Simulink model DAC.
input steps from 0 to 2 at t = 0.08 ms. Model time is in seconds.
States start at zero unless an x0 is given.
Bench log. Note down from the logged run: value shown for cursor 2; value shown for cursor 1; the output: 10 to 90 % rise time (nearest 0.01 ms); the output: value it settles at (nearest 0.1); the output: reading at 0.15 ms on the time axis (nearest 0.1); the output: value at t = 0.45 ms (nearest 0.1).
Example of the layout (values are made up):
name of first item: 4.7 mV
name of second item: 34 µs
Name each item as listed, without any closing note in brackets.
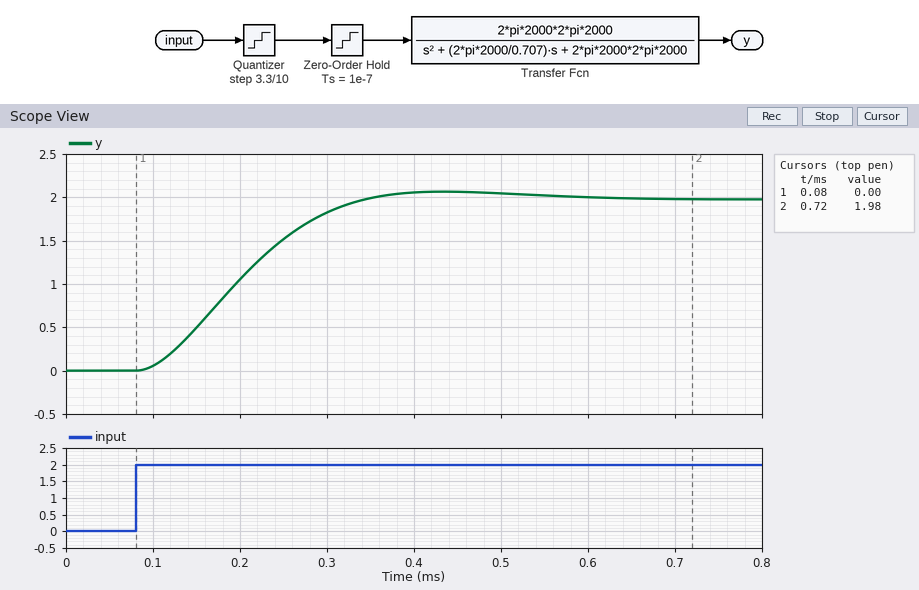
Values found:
value shown for cursor 2: 1.98
value shown for cursor 1: 0.00
the output: 10 to 90 % rise time: 0.17 ms
the output: value it settles at: 2.0
the output: reading at 0.15 ms on the time axis: 0.5
the output: value at t = 0.45 ms: 2.1
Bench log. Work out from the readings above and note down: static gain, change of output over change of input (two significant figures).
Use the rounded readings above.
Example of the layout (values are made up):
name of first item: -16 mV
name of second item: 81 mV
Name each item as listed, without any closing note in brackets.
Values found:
static gain, change of output over change of input: 1.0
